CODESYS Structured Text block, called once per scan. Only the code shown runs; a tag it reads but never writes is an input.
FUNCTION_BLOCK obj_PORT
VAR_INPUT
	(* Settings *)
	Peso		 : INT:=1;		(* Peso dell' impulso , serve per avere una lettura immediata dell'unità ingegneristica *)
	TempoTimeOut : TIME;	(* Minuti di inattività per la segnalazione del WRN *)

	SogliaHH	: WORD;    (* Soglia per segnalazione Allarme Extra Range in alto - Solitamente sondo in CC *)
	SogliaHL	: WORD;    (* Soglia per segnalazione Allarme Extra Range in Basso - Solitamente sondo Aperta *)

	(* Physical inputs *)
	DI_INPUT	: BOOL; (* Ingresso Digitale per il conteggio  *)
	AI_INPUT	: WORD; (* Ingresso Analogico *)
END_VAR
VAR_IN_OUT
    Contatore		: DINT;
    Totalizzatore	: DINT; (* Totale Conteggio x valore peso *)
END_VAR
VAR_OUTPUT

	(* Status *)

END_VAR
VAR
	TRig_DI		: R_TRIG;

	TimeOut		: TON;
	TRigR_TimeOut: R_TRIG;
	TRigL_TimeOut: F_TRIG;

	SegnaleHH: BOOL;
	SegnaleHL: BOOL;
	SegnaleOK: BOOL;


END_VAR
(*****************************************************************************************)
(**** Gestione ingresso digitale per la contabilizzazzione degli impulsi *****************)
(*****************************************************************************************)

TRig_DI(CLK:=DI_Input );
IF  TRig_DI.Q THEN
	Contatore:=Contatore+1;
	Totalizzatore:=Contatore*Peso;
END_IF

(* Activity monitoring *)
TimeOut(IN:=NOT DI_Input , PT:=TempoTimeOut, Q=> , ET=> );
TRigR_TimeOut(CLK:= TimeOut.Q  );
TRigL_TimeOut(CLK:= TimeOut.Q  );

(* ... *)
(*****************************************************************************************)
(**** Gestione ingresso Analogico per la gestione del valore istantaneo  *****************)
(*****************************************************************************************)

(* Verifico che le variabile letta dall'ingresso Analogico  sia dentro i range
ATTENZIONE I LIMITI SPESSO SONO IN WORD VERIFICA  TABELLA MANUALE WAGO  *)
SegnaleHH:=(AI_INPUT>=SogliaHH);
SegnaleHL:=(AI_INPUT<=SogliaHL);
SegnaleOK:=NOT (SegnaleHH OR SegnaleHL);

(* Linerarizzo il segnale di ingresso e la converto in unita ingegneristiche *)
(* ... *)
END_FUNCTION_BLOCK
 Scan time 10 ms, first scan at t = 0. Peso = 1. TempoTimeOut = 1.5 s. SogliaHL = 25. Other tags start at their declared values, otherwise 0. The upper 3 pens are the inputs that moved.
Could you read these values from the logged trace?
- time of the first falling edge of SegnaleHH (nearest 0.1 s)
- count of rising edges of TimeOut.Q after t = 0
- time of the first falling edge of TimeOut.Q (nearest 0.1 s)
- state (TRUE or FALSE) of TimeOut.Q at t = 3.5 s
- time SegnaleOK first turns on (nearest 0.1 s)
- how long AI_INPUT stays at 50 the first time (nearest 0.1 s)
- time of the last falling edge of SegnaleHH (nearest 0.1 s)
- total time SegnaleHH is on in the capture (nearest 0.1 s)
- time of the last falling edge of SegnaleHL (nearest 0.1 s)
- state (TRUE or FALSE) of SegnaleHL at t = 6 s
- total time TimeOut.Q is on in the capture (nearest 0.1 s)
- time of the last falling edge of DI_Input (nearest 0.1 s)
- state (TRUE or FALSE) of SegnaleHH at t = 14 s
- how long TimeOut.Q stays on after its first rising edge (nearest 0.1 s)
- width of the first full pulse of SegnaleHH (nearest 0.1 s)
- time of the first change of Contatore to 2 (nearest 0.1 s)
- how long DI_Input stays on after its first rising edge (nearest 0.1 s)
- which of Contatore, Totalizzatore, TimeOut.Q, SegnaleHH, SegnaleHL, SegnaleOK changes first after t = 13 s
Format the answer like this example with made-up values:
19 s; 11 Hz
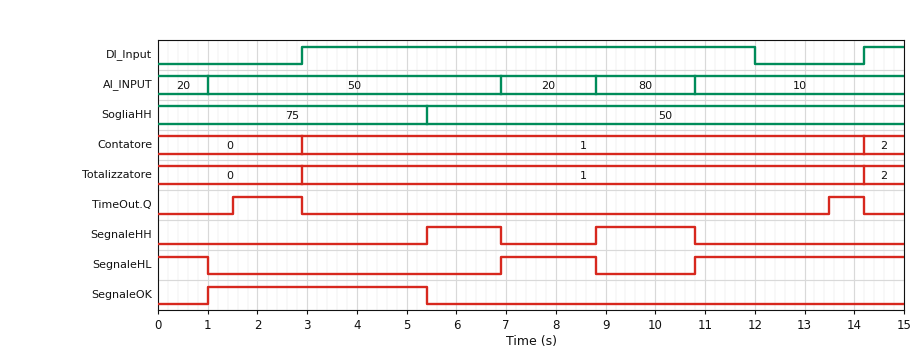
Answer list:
6.9 s; 2; 2.9 s; FALSE; 1.0 s; 5.9 s; 10.8 s; 3.5 s; 8.8 s; FALSE; 2.1 s; 12.0 s; FALSE; 1.4 s; 1.5 s; 14.2 s; 9.1 s; TimeOut.Q
